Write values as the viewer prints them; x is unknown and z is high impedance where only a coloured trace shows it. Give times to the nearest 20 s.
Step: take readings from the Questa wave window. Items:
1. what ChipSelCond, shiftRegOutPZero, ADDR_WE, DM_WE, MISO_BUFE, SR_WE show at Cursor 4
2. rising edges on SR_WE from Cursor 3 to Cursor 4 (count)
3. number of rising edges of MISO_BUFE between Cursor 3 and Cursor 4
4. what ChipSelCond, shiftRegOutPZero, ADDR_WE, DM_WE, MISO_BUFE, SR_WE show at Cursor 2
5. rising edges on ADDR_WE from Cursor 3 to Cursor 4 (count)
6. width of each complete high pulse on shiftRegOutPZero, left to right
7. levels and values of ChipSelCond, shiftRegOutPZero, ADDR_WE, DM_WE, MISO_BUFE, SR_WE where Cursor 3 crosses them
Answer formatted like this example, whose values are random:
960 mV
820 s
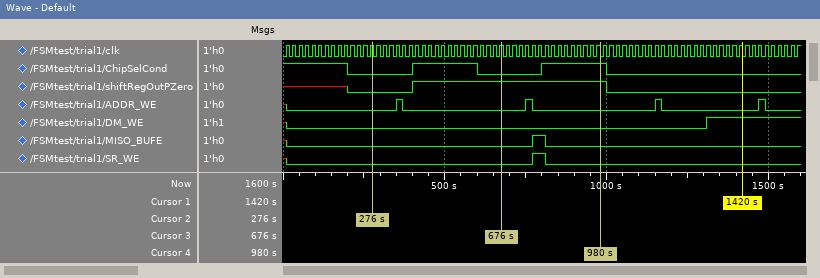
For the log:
ChipSelCond=1, shiftRegOutPZero=1, ADDR_WE=0, DM_WE=0, MISO_BUFE=0, SR_WE=0
1
1
ChipSelCond=0, shiftRegOutPZero=0, ADDR_WE=0, DM_WE=0, MISO_BUFE=0, SR_WE=0
1
600 s
ChipSelCond=0, shiftRegOutPZero=1, ADDR_WE=0, DM_WE=0, MISO_BUFE=0, SR_WE=0
